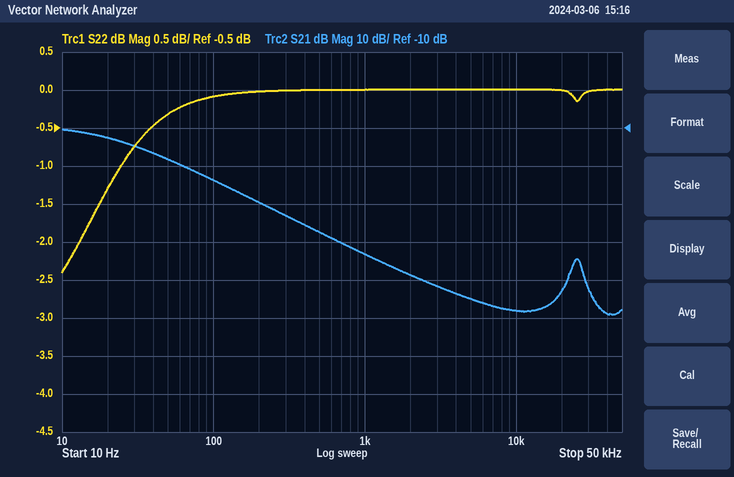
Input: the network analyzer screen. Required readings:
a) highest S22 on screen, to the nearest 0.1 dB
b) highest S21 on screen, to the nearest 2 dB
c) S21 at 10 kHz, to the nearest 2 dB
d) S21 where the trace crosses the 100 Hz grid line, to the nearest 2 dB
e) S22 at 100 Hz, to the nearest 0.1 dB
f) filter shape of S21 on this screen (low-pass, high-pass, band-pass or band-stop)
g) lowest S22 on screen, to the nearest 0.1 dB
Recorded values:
0.0 dB
-10 dB
-58 dB
-24 dB
-0.1 dB
low-pass
-2.4 dB
